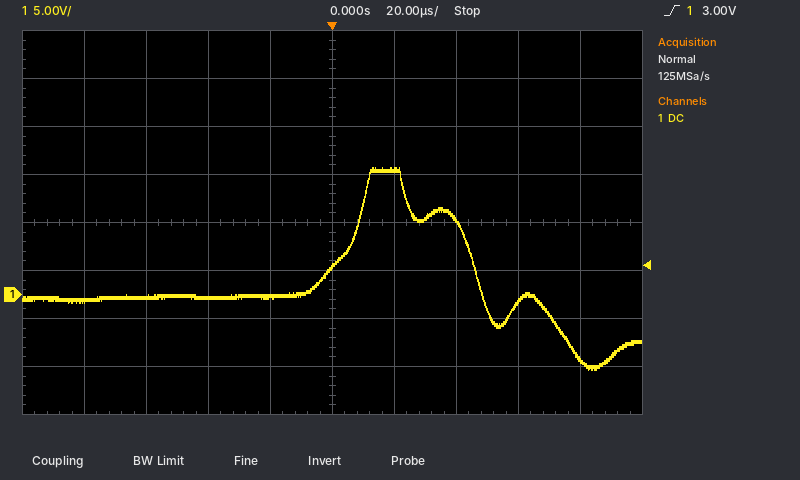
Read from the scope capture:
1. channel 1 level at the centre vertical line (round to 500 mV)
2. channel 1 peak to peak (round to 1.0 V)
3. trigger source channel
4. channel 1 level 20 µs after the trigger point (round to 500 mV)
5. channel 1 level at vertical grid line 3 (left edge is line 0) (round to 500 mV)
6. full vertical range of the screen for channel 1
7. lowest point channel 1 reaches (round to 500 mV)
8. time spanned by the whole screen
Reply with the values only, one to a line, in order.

3.0 V
21.0 V
channel 1
13.0 V
-500 mV
40 V
-8.0 V
200 µs
